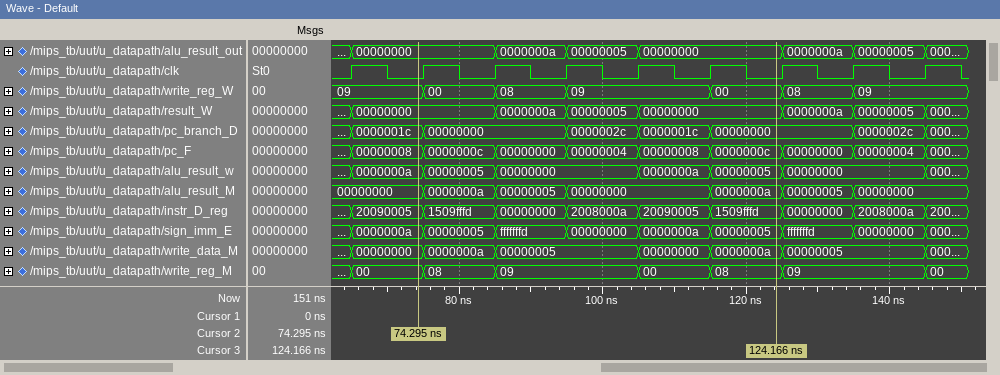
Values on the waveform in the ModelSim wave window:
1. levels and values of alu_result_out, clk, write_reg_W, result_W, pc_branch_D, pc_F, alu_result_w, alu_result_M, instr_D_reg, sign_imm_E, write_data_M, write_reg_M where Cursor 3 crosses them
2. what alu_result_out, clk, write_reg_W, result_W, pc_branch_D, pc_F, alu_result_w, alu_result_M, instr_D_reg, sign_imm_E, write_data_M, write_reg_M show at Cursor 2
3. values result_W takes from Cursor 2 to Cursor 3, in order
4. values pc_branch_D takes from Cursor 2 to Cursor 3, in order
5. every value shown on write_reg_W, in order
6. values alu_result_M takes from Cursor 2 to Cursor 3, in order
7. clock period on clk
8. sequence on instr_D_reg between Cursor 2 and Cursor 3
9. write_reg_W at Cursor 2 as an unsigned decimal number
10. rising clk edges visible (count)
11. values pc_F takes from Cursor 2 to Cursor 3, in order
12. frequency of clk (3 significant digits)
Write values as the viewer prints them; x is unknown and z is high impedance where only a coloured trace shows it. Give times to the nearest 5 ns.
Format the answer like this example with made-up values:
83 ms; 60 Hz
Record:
alu_result_out=00000000, clk=0, write_reg_W=00, result_W=00000000, pc_branch_D=00000000, pc_F=0000000c, alu_result_w=00000005, alu_result_M=0000000a, instr_D_reg=1509fffd, sign_imm_E=00000005, write_data_M=0000000a, write_reg_M=08; alu_result_out=00000000, clk=0, write_reg_W=09, result_W=00000000, pc_branch_D=0000001c, pc_F=00000008, alu_result_w=0000000a, alu_result_M=00000000, instr_D_reg=20090005, sign_imm_E=0000000a, write_data_M=00000000, write_reg_M=00; 00000000, 0000000a, 00000005, 00000000; 0000001c, 00000000, 0000002c, 0000001c, 00000000; 09, 00, 08, 09, 00, 08, 09; 00000000, 0000000a, 00000005, 00000000, 0000000a; 10 ns; 20090005, 1509fffd, 00000000, 2008000a, 20090005, 1509fffd; 9; 9; 00000008, 0000000c, 00000000, 00000004, 00000008, 0000000c; 100 MHz
